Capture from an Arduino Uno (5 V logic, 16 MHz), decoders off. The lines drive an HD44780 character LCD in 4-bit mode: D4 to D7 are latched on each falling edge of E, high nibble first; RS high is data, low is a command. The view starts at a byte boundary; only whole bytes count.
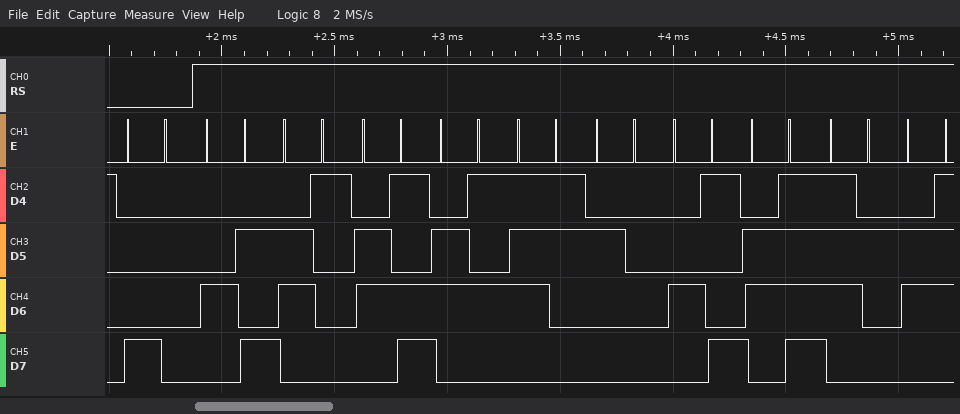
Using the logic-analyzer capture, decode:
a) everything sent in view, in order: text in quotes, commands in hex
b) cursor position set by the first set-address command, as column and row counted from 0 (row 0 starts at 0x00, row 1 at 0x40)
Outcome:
0x80 "James Iorg"
column 0, row 0
